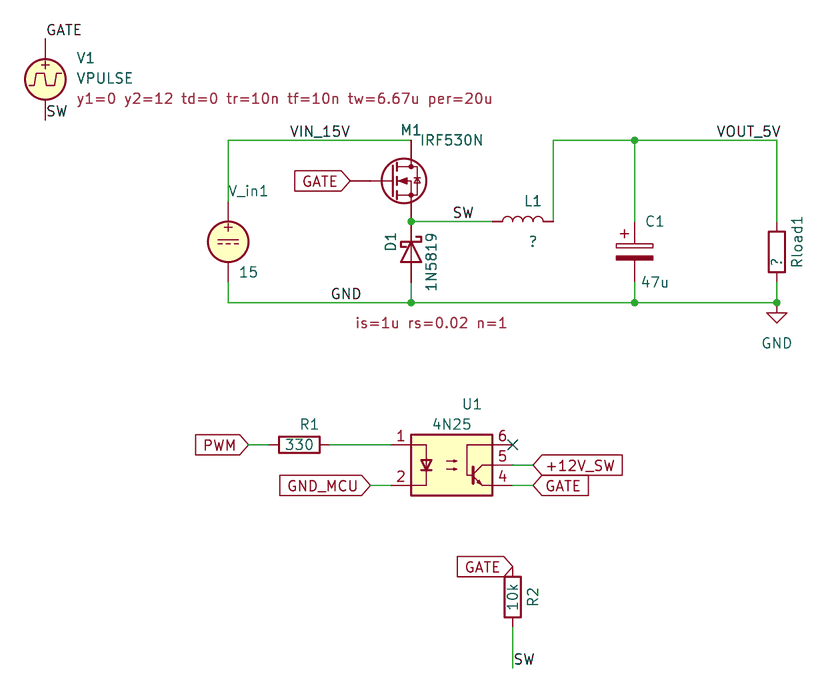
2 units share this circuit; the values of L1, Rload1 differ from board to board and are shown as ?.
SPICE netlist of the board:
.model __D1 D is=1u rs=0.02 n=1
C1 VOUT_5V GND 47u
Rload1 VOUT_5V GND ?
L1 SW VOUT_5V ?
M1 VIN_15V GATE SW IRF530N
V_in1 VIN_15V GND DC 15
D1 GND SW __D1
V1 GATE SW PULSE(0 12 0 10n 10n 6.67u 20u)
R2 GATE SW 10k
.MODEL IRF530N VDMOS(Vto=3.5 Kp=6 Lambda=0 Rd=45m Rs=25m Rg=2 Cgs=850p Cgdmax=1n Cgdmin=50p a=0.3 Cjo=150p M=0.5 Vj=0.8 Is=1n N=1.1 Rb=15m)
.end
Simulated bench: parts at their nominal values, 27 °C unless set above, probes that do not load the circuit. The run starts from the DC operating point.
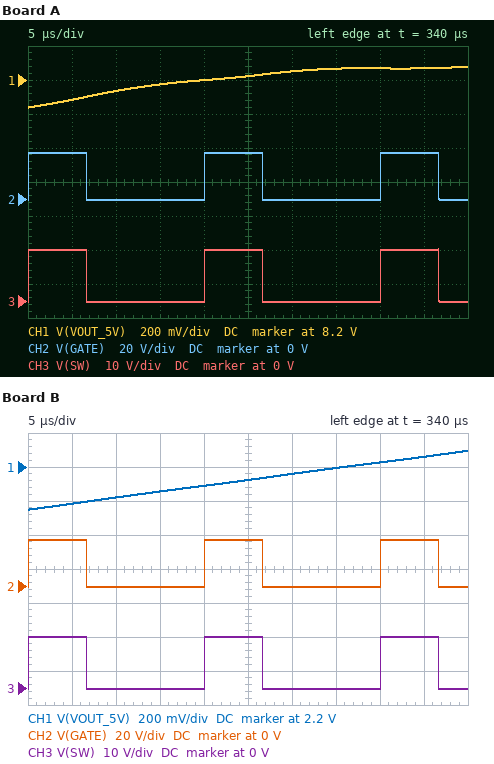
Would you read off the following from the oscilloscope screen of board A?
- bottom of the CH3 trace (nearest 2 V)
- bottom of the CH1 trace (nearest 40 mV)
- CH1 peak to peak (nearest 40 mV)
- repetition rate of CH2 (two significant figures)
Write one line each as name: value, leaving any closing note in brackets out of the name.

bottom of the CH3 trace: 0 V
bottom of the CH1 trace: 8.04 V
CH1 peak to peak: 240 mV
repetition rate of CH2: 50 kHz
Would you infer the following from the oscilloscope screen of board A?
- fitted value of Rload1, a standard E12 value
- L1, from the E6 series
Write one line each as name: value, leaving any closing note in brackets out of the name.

fitted value of Rload1, a standard E12 value: 15 Ω
L1, from the E6 series: 330 µH
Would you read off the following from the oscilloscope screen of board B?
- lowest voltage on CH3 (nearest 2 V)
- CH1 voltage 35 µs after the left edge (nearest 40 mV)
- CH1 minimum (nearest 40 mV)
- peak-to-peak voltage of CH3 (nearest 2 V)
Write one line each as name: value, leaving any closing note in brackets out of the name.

lowest voltage on CH3: 0 V
CH1 voltage 35 µs after the left edge: 2.20 V
CH1 minimum: 1.96 V
peak-to-peak voltage of CH3: 16 V
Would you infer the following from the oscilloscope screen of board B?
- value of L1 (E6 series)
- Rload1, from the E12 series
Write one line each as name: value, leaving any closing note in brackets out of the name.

value of L1: 1.5 mH
Rload1, from the E12 series: 3.3 Ω
